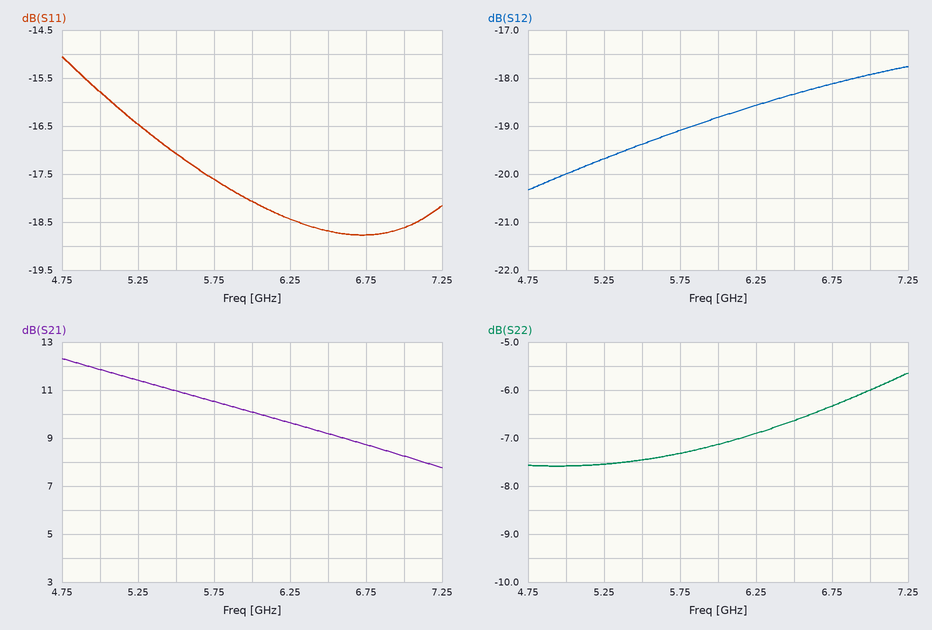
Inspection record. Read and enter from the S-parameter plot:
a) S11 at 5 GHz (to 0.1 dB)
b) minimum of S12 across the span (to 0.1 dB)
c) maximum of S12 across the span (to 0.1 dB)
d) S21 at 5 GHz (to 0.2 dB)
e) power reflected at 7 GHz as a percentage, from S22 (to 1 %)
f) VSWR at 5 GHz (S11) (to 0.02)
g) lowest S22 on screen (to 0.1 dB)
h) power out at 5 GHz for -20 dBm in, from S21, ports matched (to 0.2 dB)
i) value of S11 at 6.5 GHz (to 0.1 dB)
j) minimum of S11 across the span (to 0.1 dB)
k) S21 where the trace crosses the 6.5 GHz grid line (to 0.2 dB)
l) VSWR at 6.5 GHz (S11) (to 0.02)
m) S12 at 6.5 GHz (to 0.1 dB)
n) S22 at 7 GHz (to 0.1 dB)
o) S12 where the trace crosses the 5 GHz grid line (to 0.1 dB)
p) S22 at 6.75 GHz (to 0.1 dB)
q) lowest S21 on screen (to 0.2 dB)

-15.8 dB
-20.3 dB
-17.8 dB
11.8 dB
25 %
1.38
-7.6 dB
-8.2 dBm
-18.7 dB
-18.8 dB
9.2 dB
1.26
-18.3 dB
-6.0 dB
-20.0 dB
-6.3 dB
7.8 dB
